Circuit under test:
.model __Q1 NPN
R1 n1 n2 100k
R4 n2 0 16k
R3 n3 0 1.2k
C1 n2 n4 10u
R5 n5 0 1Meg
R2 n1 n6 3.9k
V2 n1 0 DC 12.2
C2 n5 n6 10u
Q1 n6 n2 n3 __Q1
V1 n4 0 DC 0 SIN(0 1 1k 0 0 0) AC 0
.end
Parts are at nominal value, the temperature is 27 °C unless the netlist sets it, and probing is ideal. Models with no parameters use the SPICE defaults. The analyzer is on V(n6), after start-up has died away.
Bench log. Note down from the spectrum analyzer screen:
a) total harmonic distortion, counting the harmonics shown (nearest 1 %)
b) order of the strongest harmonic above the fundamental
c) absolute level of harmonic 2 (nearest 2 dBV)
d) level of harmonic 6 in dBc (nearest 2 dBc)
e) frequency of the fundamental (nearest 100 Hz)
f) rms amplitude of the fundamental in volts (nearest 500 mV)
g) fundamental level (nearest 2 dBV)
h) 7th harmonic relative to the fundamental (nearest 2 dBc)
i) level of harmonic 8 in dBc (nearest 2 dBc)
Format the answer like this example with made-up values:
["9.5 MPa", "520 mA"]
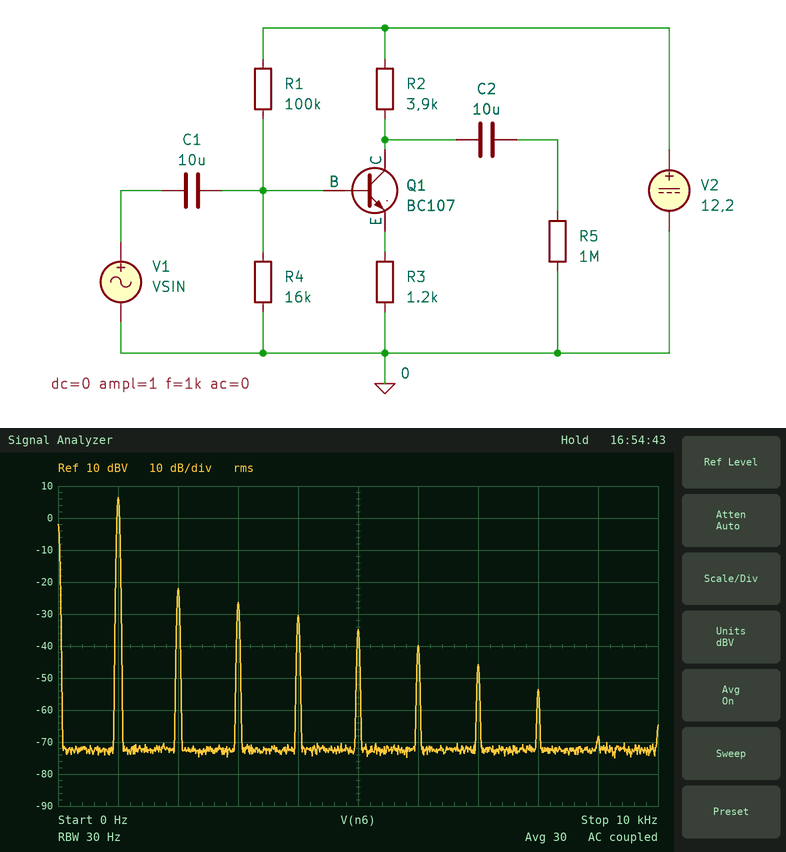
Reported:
["5 %", "2", "-22 dBV", "-46 dBc", "1.0 kHz", "2.0 V", "6 dBV", "-52 dBc", "-60 dBc"]
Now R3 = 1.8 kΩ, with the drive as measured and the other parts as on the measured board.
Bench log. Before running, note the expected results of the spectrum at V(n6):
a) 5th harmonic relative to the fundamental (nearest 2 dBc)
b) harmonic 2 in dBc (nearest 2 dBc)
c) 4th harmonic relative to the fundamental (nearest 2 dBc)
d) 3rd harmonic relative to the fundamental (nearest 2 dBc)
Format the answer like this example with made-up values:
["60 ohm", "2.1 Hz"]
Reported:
["-44 dBc", "-30 dBc", "-40 dBc", "-36 dBc"]
